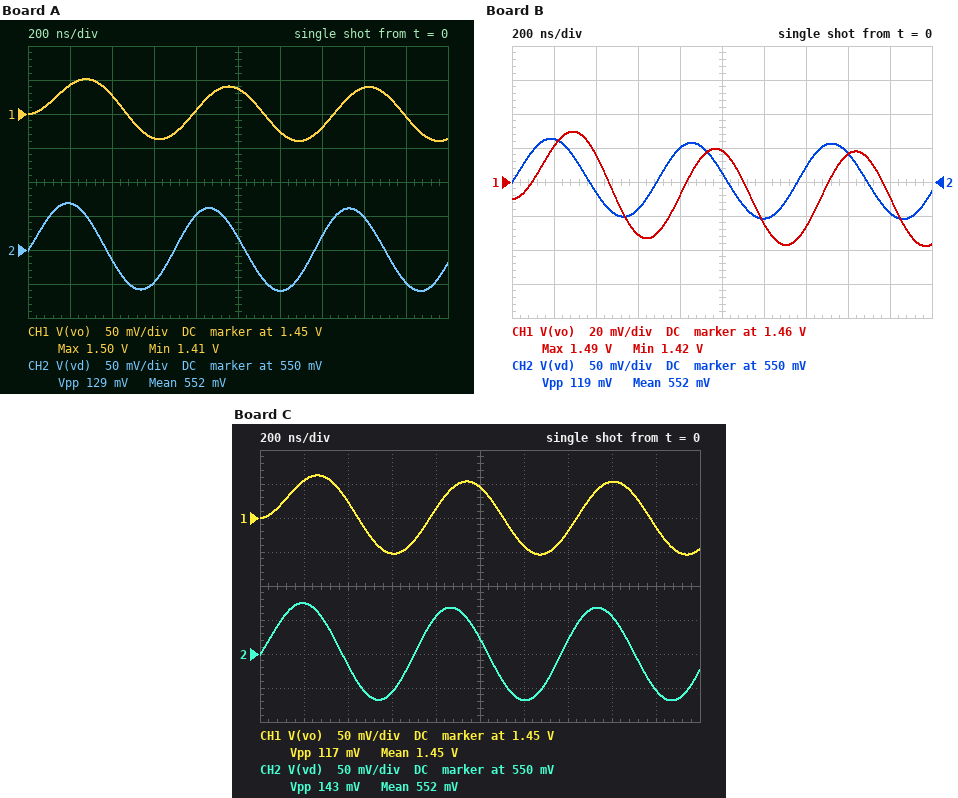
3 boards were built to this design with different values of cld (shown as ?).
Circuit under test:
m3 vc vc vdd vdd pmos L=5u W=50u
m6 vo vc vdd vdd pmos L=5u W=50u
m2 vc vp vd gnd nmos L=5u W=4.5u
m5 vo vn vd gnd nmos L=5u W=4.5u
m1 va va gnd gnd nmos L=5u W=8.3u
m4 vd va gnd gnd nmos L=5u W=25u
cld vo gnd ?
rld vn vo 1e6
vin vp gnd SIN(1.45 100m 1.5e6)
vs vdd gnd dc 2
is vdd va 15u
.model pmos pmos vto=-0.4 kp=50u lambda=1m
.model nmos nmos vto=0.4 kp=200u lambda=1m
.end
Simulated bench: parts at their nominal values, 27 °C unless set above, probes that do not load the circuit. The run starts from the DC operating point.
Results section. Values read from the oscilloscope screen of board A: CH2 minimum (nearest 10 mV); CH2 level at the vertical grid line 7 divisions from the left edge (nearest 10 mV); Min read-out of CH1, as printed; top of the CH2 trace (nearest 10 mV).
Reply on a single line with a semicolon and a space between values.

490 mV; 570 mV; 1.41 V; 620 mV
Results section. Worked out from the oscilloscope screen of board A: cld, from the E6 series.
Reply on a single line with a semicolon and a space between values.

22 pF
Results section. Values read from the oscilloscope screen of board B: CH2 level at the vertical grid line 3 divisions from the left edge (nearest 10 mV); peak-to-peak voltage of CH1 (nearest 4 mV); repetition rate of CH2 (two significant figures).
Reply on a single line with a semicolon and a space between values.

510 mV; 68 mV; 1.5 MHz
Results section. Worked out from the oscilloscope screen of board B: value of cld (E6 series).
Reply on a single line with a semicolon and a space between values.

33 pF
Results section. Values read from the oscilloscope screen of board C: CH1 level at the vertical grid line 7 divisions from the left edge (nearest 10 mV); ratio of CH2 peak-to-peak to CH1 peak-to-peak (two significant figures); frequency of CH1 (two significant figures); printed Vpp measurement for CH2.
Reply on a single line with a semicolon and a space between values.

1.43 V; 1.2; 1.5 MHz; 143 mV
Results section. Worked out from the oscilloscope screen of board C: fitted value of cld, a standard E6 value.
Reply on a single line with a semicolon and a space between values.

15 pF
